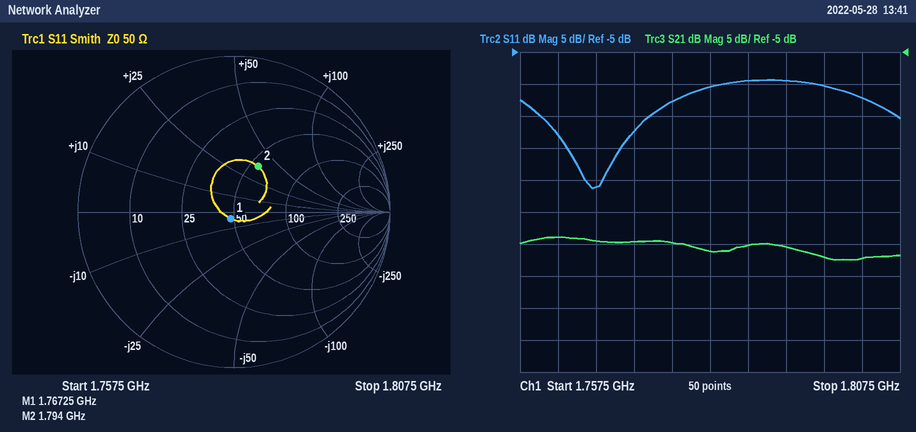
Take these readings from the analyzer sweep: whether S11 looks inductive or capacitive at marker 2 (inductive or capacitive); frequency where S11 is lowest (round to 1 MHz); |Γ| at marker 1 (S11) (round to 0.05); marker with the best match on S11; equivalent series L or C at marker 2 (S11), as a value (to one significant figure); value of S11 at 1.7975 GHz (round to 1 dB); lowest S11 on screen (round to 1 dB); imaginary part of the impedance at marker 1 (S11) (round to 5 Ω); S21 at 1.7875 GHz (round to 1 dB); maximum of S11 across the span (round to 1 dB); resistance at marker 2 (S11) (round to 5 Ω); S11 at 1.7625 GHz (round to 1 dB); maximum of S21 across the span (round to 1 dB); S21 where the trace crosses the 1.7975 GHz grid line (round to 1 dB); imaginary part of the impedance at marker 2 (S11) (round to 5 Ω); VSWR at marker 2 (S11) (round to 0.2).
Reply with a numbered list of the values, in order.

1. inductive
2. 1.767 GHz
3. 0.05
4. marker 1
5. 3 nH
6. -10 dB
7. -26 dB
8. -5 Ω
9. -35 dB
10. -9 dB
11. 55 Ω
12. -18 dB
13. -34 dB
14. -37 dB
15. +35 Ω
16. 2.0
